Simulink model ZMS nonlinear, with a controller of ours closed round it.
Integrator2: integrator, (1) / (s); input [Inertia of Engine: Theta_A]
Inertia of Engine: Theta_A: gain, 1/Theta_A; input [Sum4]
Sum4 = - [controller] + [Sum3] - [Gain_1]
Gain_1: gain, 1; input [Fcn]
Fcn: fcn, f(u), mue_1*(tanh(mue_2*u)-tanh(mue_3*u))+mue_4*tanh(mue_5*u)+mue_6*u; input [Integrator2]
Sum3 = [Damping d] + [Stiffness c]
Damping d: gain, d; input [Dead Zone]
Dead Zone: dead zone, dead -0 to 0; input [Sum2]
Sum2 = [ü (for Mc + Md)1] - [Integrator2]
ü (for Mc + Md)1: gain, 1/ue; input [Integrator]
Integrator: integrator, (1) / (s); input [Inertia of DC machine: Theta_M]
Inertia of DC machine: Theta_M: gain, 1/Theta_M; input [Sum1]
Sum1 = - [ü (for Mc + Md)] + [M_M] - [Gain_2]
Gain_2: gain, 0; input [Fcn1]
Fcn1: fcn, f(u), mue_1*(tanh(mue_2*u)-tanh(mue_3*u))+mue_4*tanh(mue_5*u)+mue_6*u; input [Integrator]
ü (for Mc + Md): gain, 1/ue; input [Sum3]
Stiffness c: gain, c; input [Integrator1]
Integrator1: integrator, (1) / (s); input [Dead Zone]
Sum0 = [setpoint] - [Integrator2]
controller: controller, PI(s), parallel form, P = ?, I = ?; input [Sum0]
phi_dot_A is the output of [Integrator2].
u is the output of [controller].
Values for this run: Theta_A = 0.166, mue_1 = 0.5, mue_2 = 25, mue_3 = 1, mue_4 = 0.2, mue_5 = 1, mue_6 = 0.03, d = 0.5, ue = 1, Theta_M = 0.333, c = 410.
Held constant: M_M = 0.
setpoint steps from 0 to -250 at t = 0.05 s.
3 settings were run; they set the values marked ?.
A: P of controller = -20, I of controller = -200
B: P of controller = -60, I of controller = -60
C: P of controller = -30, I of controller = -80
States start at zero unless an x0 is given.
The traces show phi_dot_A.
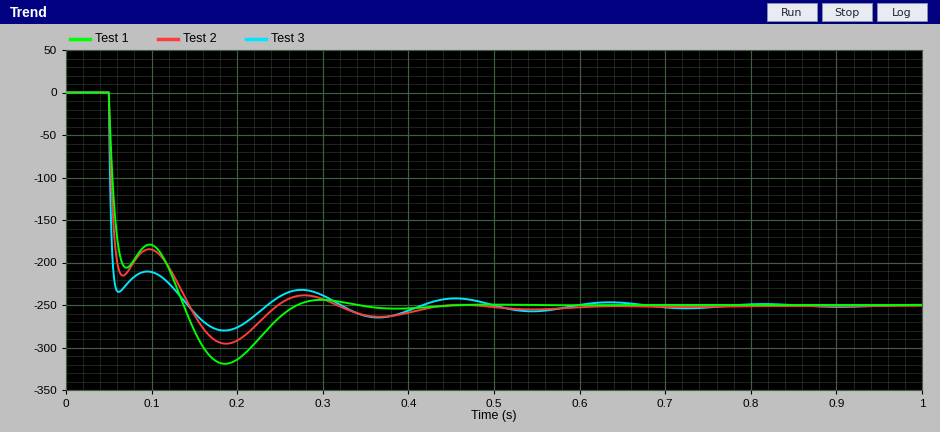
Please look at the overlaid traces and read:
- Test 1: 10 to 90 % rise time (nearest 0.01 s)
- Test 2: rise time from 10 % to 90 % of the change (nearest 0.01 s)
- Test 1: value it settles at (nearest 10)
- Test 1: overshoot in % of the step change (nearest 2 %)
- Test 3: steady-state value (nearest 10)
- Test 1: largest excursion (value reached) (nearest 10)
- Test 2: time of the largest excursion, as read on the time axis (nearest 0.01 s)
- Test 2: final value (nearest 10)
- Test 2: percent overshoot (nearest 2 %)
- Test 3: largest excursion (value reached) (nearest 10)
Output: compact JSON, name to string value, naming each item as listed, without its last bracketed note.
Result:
{"Test 1: 10 to 90 % rise time": "0.08 s", "Test 2: rise time from 10 % to 90 % of the change": "0.08 s", "Test 1: value it settles at": "-250", "Test 1: overshoot in % of the step change": "28 %", "Test 3: steady-state value": "-250", "Test 1: largest excursion (value reached)": "-320", "Test 2: time of the largest excursion, as read on the time axis": "0.19 s", "Test 2: final value": "-250", "Test 2: percent overshoot": "18 %", "Test 3: largest excursion (value reached)": "-280"}
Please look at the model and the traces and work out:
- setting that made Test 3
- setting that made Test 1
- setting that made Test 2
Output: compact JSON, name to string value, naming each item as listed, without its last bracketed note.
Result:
{"setting that made Test 3": "B", "setting that made Test 1": "A", "setting that made Test 2": "C"}
